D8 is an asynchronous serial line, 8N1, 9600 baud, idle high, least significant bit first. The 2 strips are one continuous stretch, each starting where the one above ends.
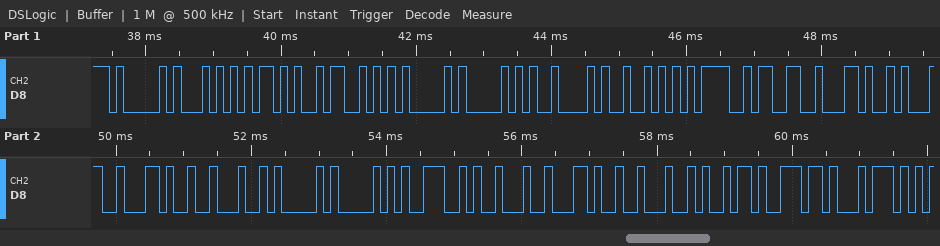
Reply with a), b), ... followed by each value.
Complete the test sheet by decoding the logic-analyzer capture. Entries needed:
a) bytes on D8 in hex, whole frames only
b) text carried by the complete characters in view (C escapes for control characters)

a) 0x41 0x54 0x2B 0x53 0x41 0x50 0x42 0x52 0x3D 0x33 0x2C 0x31 0x2C 0x22 0x41 0x50 0x4E 0x22 0x2C 0x22 0x69 0x6E 0x74
b) "AT+SAPBR=3,1,\"APN\",\"int"
